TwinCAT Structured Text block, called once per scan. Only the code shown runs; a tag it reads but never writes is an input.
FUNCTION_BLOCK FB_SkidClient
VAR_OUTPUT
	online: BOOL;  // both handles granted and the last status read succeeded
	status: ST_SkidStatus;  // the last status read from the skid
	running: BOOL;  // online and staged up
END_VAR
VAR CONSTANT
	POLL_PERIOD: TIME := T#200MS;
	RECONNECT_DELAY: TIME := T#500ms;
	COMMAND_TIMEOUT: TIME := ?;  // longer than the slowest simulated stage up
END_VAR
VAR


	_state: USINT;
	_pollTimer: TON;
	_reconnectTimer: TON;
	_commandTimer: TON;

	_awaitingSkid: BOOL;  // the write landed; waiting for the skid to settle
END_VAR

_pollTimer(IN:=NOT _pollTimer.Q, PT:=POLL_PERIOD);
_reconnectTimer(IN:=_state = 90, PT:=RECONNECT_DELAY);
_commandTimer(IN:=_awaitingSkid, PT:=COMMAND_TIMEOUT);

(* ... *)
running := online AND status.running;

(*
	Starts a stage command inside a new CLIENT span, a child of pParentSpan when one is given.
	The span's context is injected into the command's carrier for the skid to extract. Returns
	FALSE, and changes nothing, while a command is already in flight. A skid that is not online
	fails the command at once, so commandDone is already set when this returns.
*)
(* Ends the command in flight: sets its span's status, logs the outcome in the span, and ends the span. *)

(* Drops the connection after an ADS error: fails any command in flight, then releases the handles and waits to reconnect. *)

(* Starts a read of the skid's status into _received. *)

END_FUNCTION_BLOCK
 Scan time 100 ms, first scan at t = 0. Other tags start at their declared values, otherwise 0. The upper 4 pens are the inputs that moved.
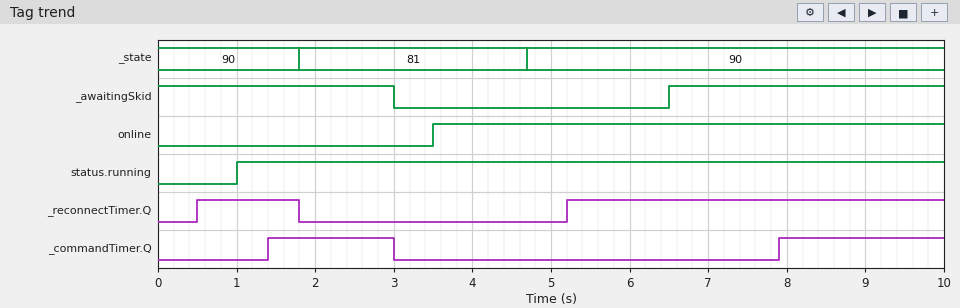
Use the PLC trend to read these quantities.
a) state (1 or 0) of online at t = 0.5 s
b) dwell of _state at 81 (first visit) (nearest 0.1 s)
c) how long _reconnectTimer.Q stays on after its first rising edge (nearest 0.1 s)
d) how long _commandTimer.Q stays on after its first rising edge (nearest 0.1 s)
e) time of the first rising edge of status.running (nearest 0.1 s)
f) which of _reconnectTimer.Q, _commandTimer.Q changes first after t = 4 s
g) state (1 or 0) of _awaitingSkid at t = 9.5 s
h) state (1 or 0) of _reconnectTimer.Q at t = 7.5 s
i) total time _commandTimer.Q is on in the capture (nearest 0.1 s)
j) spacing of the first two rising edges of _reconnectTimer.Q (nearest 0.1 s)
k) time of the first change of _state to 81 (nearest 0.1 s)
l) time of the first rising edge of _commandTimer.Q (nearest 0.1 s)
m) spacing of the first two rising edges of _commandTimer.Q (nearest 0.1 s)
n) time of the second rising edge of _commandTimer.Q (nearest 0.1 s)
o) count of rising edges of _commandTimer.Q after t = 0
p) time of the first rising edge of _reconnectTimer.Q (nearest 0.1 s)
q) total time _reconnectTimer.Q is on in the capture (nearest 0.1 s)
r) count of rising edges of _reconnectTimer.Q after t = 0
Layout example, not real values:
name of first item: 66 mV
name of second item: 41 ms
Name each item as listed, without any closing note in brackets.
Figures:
state (1 or 0) of online at t = 0.5 s: 0
dwell of _state at 81 (first visit): 2.9 s
how long _reconnectTimer.Q stays on after its first rising edge: 1.3 s
how long _commandTimer.Q stays on after its first rising edge: 1.6 s
time of the first rising edge of status.running: 1.0 s
which of _reconnectTimer.Q, _commandTimer.Q changes first after t = 4 s: _reconnectTimer.Q
state (1 or 0) of _awaitingSkid at t = 9.5 s: 1
state (1 or 0) of _reconnectTimer.Q at t = 7.5 s: 1
total time _commandTimer.Q is on in the capture: 3.7 s
spacing of the first two rising edges of _reconnectTimer.Q: 4.7 s
time of the first change of _state to 81: 1.8 s
time of the first rising edge of _commandTimer.Q: 1.4 s
spacing of the first two rising edges of _commandTimer.Q: 6.5 s
time of the second rising edge of _commandTimer.Q: 7.9 s
count of rising edges of _commandTimer.Q after t = 0: 2
time of the first rising edge of _reconnectTimer.Q: 0.5 s
total time _reconnectTimer.Q is on in the capture: 6.1 s
count of rising edges of _reconnectTimer.Q after t = 0: 2
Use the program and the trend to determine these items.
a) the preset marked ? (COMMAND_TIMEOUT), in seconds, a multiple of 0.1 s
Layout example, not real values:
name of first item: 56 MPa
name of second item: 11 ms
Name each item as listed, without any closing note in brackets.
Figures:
the preset marked ? (COMMAND_TIMEOUT), in seconds, a multiple of 0.1 s: 1.4 s
